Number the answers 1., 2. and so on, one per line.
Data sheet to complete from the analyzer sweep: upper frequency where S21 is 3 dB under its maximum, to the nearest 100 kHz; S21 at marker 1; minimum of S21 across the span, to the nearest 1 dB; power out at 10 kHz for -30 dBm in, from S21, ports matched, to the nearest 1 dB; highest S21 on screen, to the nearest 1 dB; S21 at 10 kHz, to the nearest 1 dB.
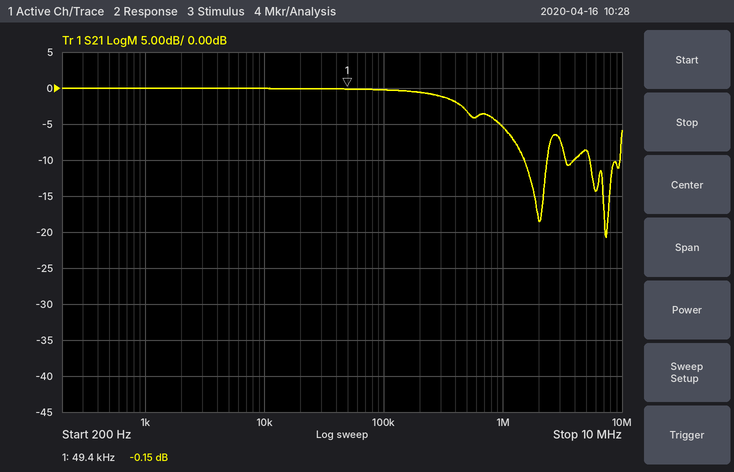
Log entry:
1. 500 kHz
2. -0.15 dB
3. -21 dB
4. -30 dBm
5. 0 dB
6. 0 dB
